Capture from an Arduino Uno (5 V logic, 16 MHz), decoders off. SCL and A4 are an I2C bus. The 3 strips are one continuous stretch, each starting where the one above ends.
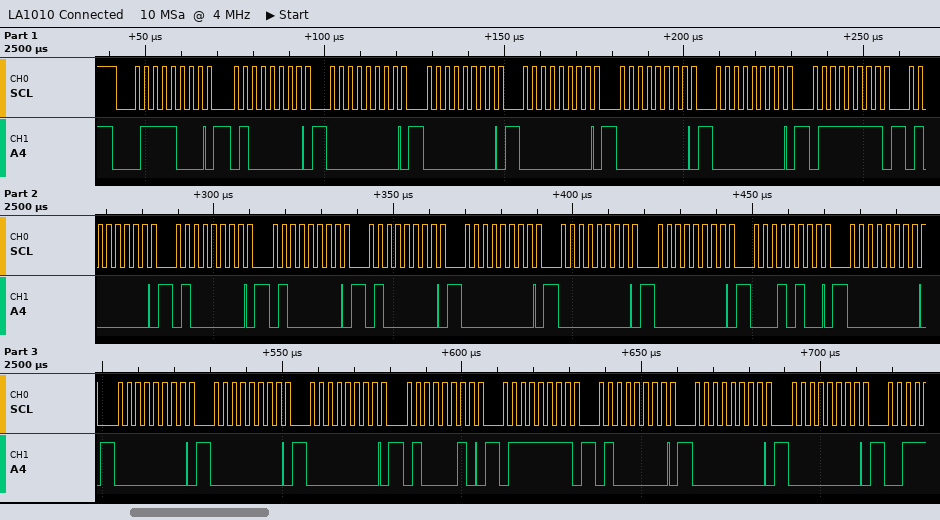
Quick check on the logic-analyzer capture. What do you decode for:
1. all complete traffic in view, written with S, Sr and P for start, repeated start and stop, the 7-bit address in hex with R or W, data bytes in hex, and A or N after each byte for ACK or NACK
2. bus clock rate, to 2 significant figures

S 3CW A 40 A 00 A 00 A 00 A 00 A 00 A 7F A 40 A 40 A 40 A 40 A 00 A 00 A 00 A 14 A 00 A 00 A 00 A 00 A 42 A 7F A 40 A 00 A 00 A
400 kHz
